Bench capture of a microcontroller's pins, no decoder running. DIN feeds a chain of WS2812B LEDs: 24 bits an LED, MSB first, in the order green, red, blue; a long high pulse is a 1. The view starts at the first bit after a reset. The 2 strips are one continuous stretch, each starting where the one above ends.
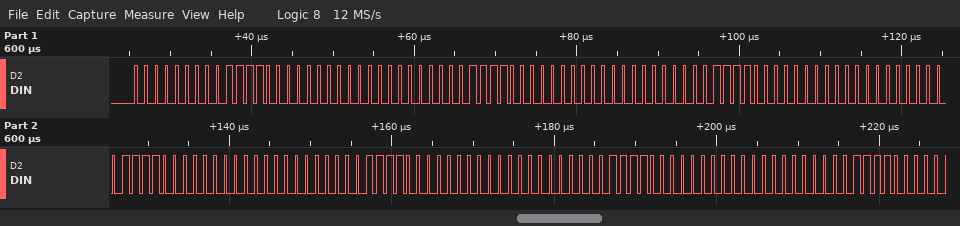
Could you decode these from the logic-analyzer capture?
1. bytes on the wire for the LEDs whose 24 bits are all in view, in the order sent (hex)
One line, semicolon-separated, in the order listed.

00 78 00 00 78 00 00 78 00 00 78 00 00 78 00 00 78 00
